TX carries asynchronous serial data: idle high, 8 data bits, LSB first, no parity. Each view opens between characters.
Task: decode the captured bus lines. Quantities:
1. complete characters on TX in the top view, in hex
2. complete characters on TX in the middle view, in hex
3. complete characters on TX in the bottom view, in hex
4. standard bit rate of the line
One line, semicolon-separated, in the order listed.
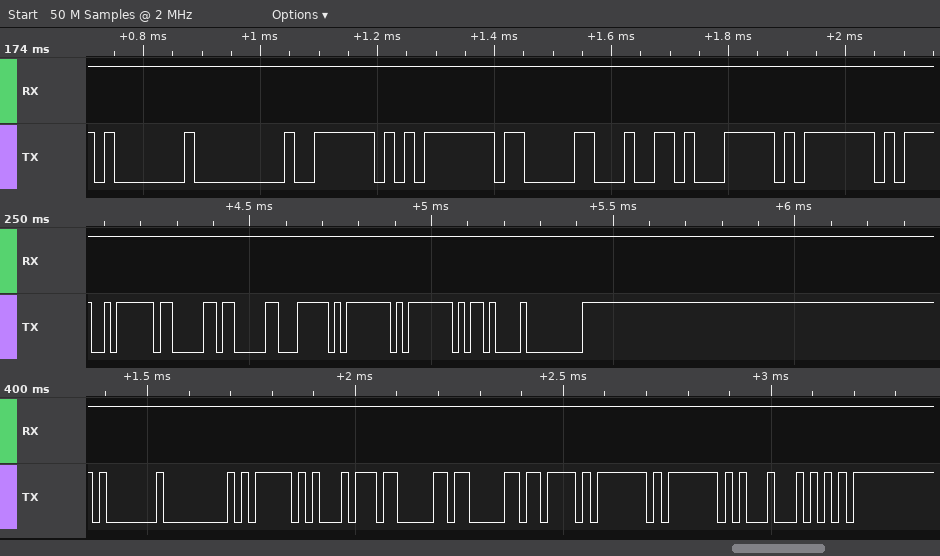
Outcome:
01, 00, 7E, FD, 83, 64, 7C, 7F; FA, 83, 83, 7C, 7F, 7F, 0B, 00; 01, 00, 7D, D1, 83, 83, 7B, 7F, 7F, 11, D5; 57600 baud
